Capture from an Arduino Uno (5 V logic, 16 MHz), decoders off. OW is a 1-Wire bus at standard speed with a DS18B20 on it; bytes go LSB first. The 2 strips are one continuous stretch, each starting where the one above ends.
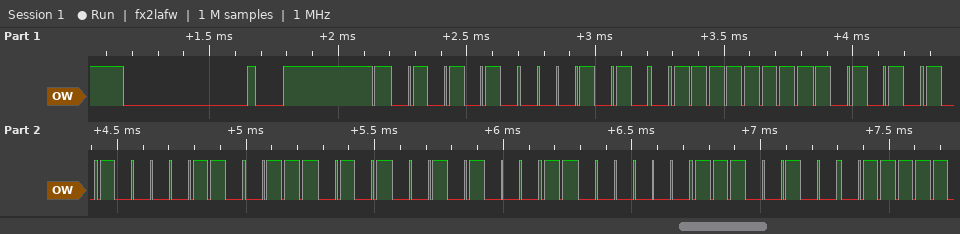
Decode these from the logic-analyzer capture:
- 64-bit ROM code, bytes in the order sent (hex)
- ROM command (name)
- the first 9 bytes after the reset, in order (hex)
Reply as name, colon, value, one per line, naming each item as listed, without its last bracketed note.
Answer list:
64-bit ROM code, bytes in the order sent: 28 FF 55 61 AE 14 03 27
ROM command: Match ROM
the first 9 bytes after the reset, in order: 55 28 FF 55 61 AE 14 03 27
